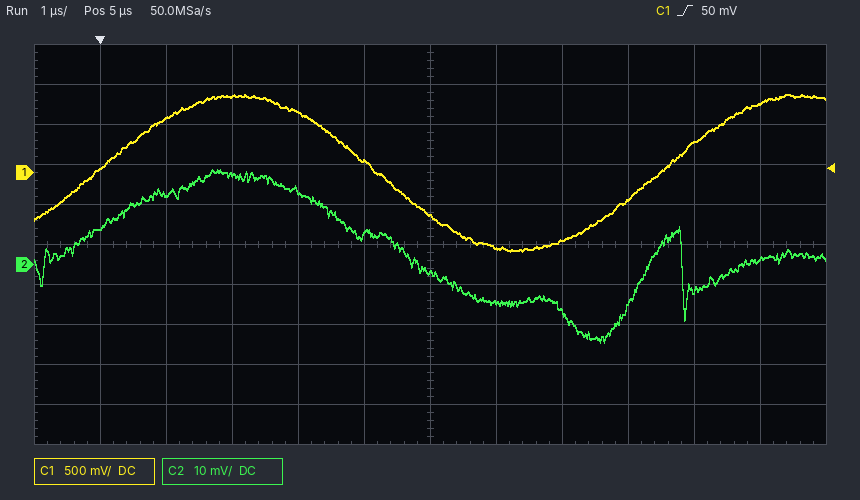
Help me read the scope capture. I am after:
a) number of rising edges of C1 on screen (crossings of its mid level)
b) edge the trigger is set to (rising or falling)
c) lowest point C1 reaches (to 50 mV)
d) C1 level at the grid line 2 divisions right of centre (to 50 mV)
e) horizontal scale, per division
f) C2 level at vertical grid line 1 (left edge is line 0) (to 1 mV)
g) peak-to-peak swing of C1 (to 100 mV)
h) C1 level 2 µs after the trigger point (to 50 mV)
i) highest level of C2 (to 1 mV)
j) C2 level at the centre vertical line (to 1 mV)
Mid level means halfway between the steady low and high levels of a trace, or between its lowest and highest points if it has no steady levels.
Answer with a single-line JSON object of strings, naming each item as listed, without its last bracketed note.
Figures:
{"number of rising edges of C1 on screen": "2", "edge the trigger is set to": "rising", "lowest point C1 reaches": "-1.00 V", "C1 level at the grid line 2 divisions right of centre": "-850 mV", "horizontal scale, per division": "1 µs", "C2 level at vertical grid line 1 (left edge is line 0)": "9 mV", "peak-to-peak swing of C1": "2.00 V", "C1 level 2 µs after the trigger point": "950 mV", "highest level of C2": "24 mV", "C2 level at the centre vertical line": "-2 mV"}
